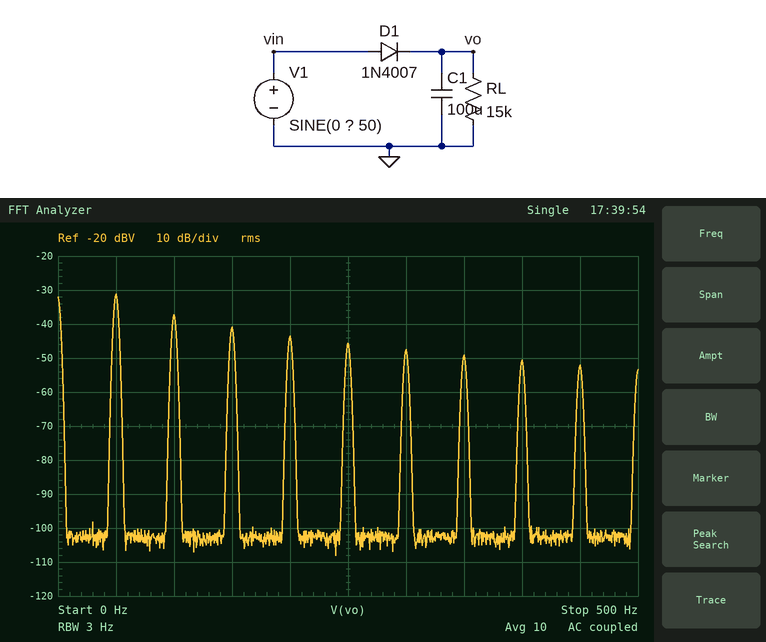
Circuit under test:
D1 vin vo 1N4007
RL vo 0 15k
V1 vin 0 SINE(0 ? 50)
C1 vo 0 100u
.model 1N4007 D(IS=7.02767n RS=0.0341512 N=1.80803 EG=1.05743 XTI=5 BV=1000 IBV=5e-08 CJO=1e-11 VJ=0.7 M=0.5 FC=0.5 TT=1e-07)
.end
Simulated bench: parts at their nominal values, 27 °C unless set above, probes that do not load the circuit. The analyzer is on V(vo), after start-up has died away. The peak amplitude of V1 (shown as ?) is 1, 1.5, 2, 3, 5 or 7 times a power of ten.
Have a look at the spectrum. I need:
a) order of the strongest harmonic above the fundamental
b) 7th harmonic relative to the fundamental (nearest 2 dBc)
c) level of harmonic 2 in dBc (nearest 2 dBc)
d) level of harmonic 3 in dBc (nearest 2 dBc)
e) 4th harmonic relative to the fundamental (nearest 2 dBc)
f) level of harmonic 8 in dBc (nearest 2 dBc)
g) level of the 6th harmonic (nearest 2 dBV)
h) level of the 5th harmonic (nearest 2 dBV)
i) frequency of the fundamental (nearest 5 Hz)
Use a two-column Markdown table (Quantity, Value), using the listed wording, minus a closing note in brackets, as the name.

| Quantity | Value |
|---|---|
| order of the strongest harmonic above the fundamental | 2 |
| 7th harmonic relative to the fundamental | -18 dBc |
| level of harmonic 2 in dBc | -6 dBc |
| level of harmonic 3 in dBc | -10 dBc |
| 4th harmonic relative to the fundamental | -12 dBc |
| level of harmonic 8 in dBc | -20 dBc |
| level of the 6th harmonic | -48 dBV |
| level of the 5th harmonic | -46 dBV |
| frequency of the fundamental | 50 Hz |
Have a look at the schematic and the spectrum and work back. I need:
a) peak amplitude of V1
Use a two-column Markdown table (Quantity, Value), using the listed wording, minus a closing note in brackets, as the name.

| Quantity | Value |
|---|---|
| peak amplitude of V1 | 10 V |
